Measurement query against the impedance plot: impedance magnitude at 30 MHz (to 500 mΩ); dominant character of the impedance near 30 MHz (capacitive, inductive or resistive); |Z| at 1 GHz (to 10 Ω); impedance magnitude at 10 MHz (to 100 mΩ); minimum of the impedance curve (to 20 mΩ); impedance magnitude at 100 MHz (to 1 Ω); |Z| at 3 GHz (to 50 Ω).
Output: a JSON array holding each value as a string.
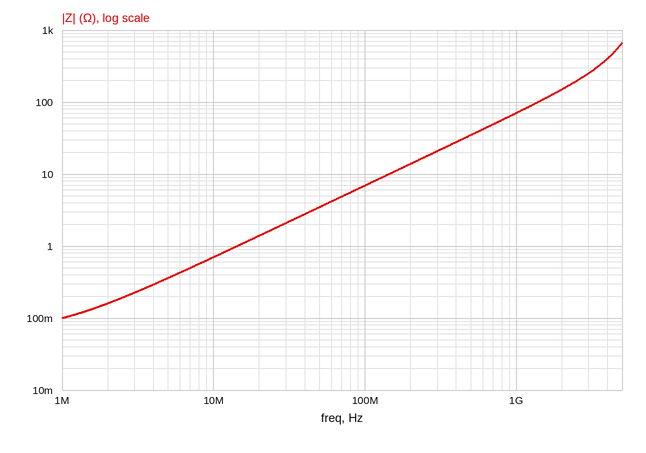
["2.0 Ω", "inductive", "70 Ω", "700 mΩ", "100 mΩ", "7 Ω", "250 Ω"]
